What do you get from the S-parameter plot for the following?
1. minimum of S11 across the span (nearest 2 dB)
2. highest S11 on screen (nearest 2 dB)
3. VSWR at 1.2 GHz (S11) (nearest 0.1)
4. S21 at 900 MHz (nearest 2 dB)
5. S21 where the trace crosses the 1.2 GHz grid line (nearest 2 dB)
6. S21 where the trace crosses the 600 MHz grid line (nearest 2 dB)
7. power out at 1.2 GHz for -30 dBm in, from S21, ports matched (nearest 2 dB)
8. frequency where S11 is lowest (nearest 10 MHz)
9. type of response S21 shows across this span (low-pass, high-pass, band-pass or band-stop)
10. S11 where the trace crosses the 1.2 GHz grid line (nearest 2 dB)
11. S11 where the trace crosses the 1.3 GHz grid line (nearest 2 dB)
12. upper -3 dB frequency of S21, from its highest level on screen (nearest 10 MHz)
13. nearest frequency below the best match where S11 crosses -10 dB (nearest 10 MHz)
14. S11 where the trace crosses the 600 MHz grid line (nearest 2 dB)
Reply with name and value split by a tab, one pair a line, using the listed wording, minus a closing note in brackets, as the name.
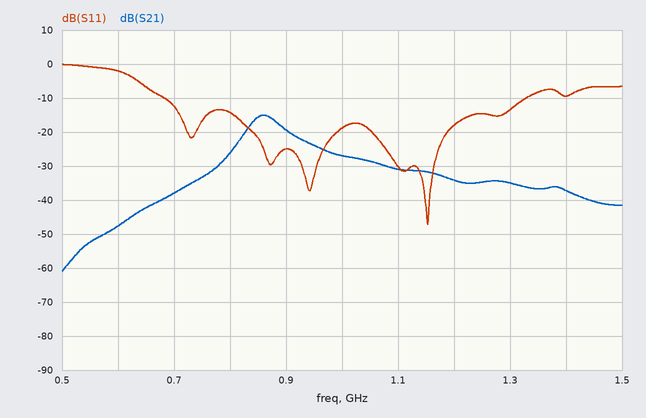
minimum of S11 across the span	-48 dB
highest S11 on screen	0 dB
VSWR at 1.2 GHz (S11)	1.3
S21 at 900 MHz	-20 dB
S21 where the trace crosses the 1.2 GHz grid line	-34 dB
S21 where the trace crosses the 600 MHz grid line	-48 dB
power out at 1.2 GHz for -30 dBm in, from S21, ports matched	-64 dBm
frequency where S11 is lowest	1.15 GHz
type of response S21 shows across this span	band-pass
S11 where the trace crosses the 1.2 GHz grid line	-18 dB
S11 where the trace crosses the 1.3 GHz grid line	-14 dB
upper -3 dB frequency of S21, from its highest level on screen	890 MHz
nearest frequency below the best match where S11 crosses -10 dB	680 MHz
S11 where the trace crosses the 600 MHz grid line	-2 dB
